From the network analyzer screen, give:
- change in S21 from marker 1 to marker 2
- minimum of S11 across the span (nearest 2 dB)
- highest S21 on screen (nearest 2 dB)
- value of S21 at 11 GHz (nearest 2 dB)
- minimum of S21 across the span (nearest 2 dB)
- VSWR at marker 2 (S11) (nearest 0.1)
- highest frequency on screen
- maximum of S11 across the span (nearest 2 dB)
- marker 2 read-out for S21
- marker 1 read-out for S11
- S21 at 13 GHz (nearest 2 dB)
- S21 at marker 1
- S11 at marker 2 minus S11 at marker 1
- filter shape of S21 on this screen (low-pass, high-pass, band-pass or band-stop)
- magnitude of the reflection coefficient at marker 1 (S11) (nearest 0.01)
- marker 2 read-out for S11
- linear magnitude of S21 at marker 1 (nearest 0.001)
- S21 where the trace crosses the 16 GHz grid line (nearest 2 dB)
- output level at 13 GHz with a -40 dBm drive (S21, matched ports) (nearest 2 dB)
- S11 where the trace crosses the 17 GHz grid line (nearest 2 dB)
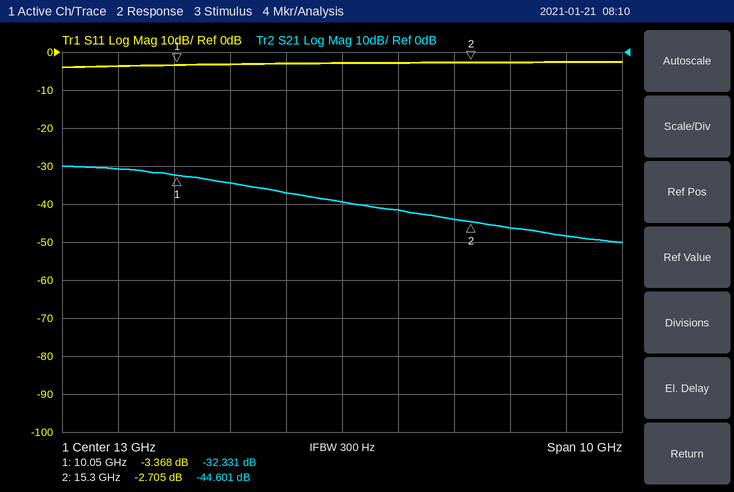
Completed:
-12.270 dB
-4 dB
-30 dB
-34 dB
-50 dB
6.5
18 GHz
-2 dB
-44.601 dB
-3.368 dB
-40 dB
-32.331 dB
0.663 dB
low-pass
0.68
-2.705 dB
0.024
-46 dB
-80 dBm
-2 dB
